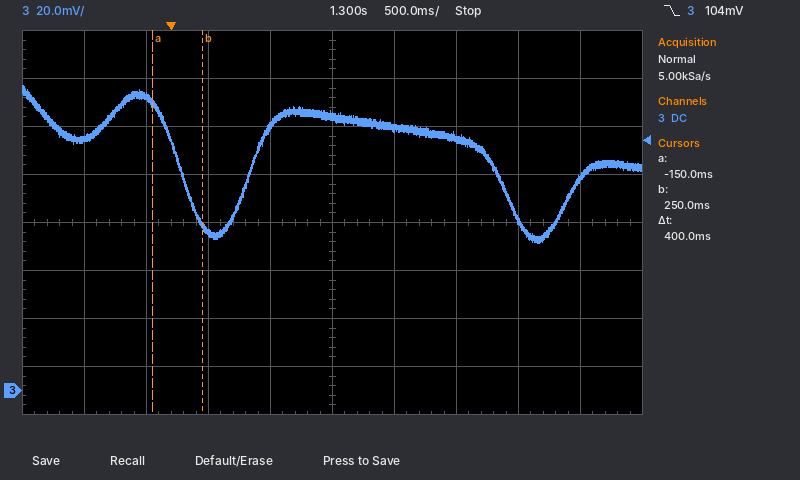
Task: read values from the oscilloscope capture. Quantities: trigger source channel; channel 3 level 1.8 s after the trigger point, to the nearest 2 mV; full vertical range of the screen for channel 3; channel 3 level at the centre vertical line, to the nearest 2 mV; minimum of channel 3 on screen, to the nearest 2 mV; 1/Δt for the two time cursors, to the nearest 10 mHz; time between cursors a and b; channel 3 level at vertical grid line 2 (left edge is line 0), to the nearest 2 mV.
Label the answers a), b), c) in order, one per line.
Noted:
a) channel 3
b) 110 mV
c) 160 mV
d) 114 mV
e) 62 mV
f) 2.50 Hz
g) 400 ms
h) 122 mV
